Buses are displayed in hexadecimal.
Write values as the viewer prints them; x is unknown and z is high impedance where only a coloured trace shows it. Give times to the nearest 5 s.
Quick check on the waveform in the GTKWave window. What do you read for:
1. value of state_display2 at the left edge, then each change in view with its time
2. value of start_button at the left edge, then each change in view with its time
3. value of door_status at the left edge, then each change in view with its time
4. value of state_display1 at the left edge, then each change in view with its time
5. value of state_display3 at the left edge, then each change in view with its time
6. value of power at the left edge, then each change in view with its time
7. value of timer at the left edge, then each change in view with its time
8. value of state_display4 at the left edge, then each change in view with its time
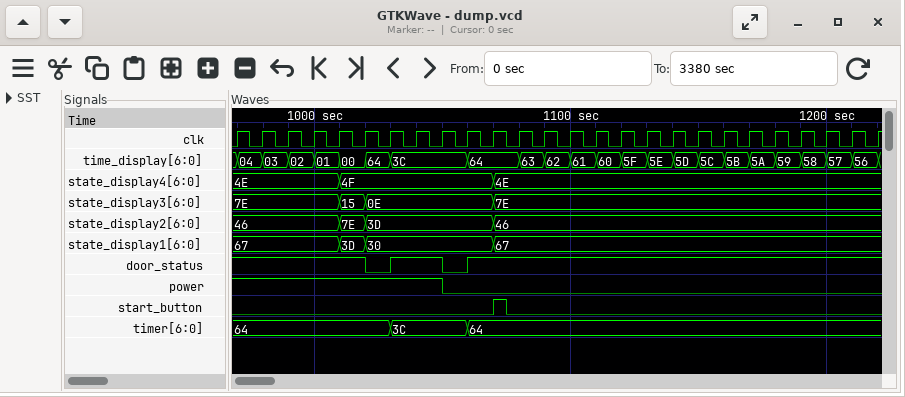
46, 7E at 1010 s, 3D at 1020 s, 46 at 1070 s
0, 1 at 1070 s, 0 at 1075 s
1, 0 at 1020 s, 1 at 1030 s, 0 at 1050 s, 1 at 1060 s
67, 3D at 1010 s, 30 at 1020 s, 67 at 1070 s
7E, 15 at 1010 s, 0E at 1020 s, 7E at 1070 s
1, 0 at 1050 s
64, 3C at 1030 s, 64 at 1060 s
4E, 4F at 1010 s, 4E at 1070 s
